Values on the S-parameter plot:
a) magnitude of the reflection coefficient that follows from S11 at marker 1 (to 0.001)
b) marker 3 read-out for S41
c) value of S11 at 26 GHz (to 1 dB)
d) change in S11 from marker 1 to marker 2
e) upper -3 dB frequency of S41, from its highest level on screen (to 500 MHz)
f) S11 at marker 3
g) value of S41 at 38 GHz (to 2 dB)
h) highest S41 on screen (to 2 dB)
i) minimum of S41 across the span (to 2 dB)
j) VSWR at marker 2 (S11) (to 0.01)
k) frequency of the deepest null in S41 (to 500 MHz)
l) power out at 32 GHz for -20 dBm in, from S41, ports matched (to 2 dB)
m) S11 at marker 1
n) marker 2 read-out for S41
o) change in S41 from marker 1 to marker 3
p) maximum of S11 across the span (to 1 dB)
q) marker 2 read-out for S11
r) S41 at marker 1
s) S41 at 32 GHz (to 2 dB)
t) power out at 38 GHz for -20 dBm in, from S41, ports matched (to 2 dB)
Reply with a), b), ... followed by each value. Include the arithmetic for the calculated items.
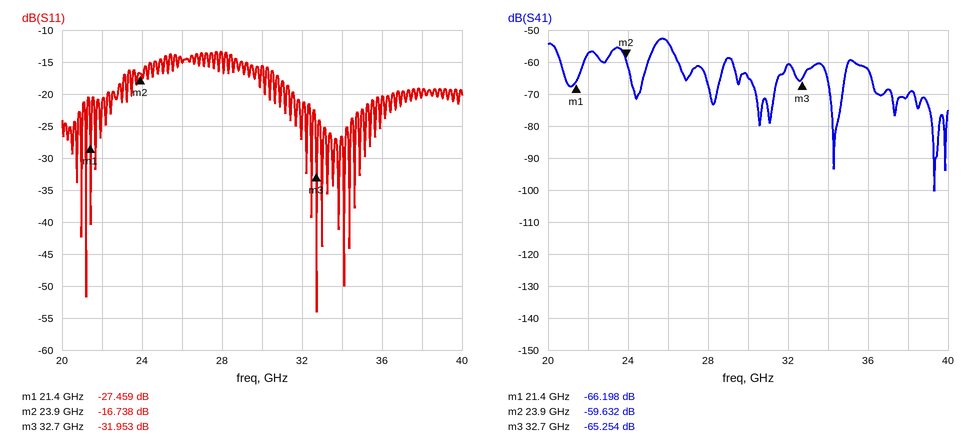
a) 10^(-27.459/20) ≈ 0.042
b) -65.254 dB
c) -15 dB
d) -16.738 − (-27.459) = 10.721 dB
e) 26.0 GHz
f) -31.953 dB
g) -70 dB
h) -52 dB
i) -100 dB
j) (1 + 0.1456)/(1 − 0.1456) ≈ 1.34
k) 39.5 GHz
l) -20 dBm + (-60 dB) = -80 dBm
m) -27.459 dB
n) -59.632 dB
o) -65.254 − (-66.198) = 0.944 dB
p) -13 dB
q) -16.738 dB
r) -66.198 dB
s) -60 dB
t) -20 dBm + (-70 dB) = -90 dBm
